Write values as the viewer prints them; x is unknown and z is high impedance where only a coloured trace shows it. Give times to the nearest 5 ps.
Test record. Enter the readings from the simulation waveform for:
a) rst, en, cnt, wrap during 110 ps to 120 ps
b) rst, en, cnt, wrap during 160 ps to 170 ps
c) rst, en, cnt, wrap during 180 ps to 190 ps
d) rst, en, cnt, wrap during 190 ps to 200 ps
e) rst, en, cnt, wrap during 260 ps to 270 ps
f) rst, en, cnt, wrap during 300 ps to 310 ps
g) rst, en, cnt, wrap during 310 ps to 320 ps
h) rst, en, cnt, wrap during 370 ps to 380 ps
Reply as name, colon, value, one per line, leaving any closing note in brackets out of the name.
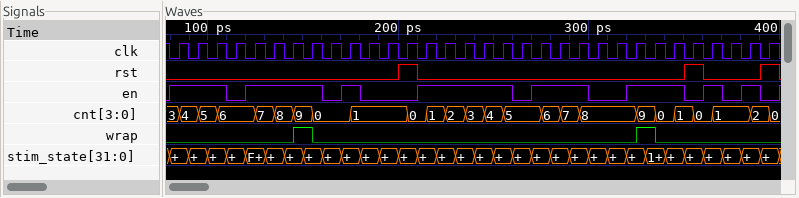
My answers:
rst, en, cnt, wrap during 110 ps to 120 ps: rst=0, en=0, cnt=6, wrap=0
rst, en, cnt, wrap during 160 ps to 170 ps: rst=0, en=0, cnt=0, wrap=0
rst, en, cnt, wrap during 180 ps to 190 ps: rst=0, en=0, cnt=1, wrap=0
rst, en, cnt, wrap during 190 ps to 200 ps: rst=0, en=0, cnt=1, wrap=0
rst, en, cnt, wrap during 260 ps to 270 ps: rst=0, en=0, cnt=5, wrap=0
rst, en, cnt, wrap during 300 ps to 310 ps: rst=0, en=0, cnt=8, wrap=0
rst, en, cnt, wrap during 310 ps to 320 ps: rst=0, en=0, cnt=8, wrap=0
rst, en, cnt, wrap during 370 ps to 380 ps: rst=0, en=0, cnt=1, wrap=0
